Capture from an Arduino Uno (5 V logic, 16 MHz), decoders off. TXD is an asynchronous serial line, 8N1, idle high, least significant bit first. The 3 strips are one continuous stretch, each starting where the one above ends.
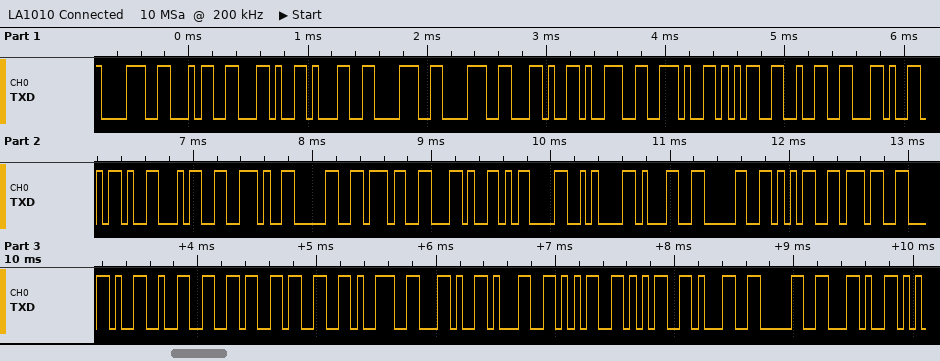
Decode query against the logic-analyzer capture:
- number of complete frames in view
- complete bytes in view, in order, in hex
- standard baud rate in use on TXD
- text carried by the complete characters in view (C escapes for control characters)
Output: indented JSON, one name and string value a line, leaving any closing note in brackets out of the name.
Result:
{
  "number of complete frames in view": "36",
  "complete bytes in view, in order, in hex": "0x38 0x34 0x2C 0x31 0x38 0x38 0x2C 0x39 0x2E 0x35 0x32 0x2C 0x2D 0x34 0x2E 0x30 0x37 0x2C 0x0D 0x0A 0x31 0x30 0x35 0x37 0x2C 0x32 0x36 0x33 0x39 0x2C 0x31 0x35 0x35 0x31 0x30 0x2C",
  "standard baud rate in use on TXD": "19200 baud",
  "text carried by the complete characters in view": "\"84,188,9.52,-4.07,\\r\\n1057,2639,15510,\""
}
